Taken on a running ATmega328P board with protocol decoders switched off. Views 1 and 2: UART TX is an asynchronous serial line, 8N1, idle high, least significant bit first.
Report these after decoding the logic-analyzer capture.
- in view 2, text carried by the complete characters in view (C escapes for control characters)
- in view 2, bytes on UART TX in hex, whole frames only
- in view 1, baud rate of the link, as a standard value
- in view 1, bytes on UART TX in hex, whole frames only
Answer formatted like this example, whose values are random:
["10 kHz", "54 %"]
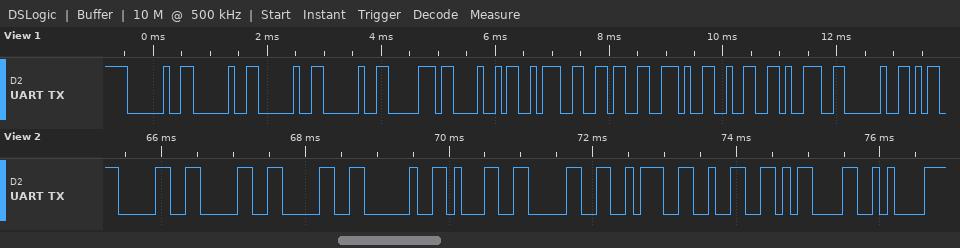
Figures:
["\"000 10:2\\r\\n\"", "0x30 0x30 0x30 0x20 0x31 0x30 0x3A 0x32 0x0D 0x0A", "9600 baud", "20 20 20 20 70 48 3A 36 2E 32 39 20"]
